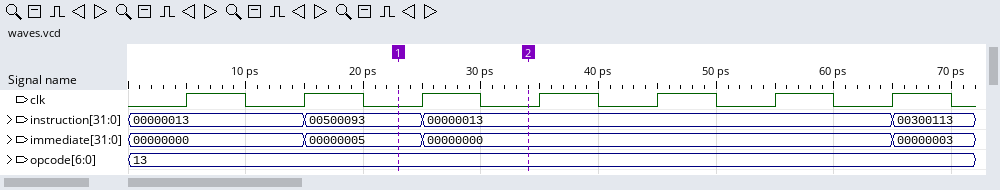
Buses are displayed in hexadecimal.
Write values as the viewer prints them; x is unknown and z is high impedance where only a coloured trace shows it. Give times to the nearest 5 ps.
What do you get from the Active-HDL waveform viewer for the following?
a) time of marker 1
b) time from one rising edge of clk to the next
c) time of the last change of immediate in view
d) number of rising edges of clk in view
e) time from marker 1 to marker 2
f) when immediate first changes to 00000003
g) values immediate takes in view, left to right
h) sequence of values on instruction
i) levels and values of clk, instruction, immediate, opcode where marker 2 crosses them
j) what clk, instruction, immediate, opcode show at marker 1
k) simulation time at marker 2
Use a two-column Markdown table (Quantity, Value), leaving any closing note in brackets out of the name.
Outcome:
| Quantity | Value |
|---|---|
| time of marker 1 | 25 ps |
| time from one rising edge of clk to the next | 10 ps |
| time of the last change of immediate in view | 65 ps |
| number of rising edges of clk in view | 7 |
| time from marker 1 to marker 2 | 10 ps |
| when immediate first changes to 00000003 | 65 ps |
| values immediate takes in view, left to right | 00000000, 00000005, 00000000, 00000003 |
| sequence of values on instruction | 00000013, 00500093, 00000013, 00300113 |
| levels and values of clk, instruction, immediate, opcode where marker 2 crosses them | clk=0, instruction=00000013, immediate=00000000, opcode=13 |
| what clk, instruction, immediate, opcode show at marker 1 | clk=0, instruction=00500093, immediate=00000005, opcode=13 |
| simulation time at marker 2 | 35 ps |
